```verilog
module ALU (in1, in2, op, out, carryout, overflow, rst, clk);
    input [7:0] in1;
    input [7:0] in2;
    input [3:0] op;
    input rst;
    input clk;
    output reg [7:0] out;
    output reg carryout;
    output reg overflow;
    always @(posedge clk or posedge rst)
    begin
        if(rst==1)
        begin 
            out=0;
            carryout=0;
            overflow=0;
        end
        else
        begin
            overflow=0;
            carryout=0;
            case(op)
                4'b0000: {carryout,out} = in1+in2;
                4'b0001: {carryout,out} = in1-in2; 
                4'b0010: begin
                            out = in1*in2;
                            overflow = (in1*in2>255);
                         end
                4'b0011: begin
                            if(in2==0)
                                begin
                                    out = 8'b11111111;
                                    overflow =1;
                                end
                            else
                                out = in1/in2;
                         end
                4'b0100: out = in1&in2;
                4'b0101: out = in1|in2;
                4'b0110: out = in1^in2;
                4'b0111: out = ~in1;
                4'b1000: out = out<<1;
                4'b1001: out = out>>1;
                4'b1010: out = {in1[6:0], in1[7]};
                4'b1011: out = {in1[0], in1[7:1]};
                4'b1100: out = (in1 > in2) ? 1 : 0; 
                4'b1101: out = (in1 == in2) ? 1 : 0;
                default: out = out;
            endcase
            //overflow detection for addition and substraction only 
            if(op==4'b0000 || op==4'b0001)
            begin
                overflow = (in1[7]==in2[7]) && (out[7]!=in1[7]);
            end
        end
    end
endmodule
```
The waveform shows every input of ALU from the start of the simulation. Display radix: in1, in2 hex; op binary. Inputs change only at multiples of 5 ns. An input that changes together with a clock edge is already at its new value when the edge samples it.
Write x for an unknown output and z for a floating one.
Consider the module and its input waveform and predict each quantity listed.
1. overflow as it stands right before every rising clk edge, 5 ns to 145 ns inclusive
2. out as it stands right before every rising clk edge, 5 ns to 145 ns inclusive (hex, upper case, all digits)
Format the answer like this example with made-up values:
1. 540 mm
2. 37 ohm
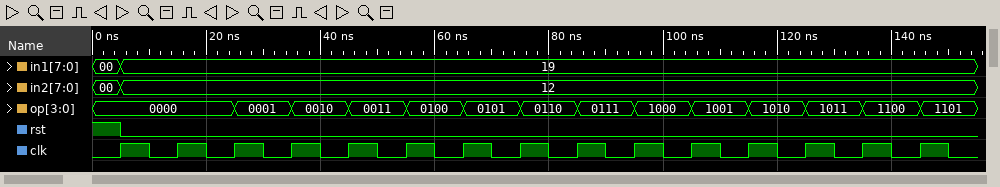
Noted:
1. 0 0 0 0 1 0 0 0 0 0 0 0 0 0 0
2. 00, 2B, 2B, 07, C2, 01, 10, 1B, 0B, E6, CC, 66, 32, 8C, 01
